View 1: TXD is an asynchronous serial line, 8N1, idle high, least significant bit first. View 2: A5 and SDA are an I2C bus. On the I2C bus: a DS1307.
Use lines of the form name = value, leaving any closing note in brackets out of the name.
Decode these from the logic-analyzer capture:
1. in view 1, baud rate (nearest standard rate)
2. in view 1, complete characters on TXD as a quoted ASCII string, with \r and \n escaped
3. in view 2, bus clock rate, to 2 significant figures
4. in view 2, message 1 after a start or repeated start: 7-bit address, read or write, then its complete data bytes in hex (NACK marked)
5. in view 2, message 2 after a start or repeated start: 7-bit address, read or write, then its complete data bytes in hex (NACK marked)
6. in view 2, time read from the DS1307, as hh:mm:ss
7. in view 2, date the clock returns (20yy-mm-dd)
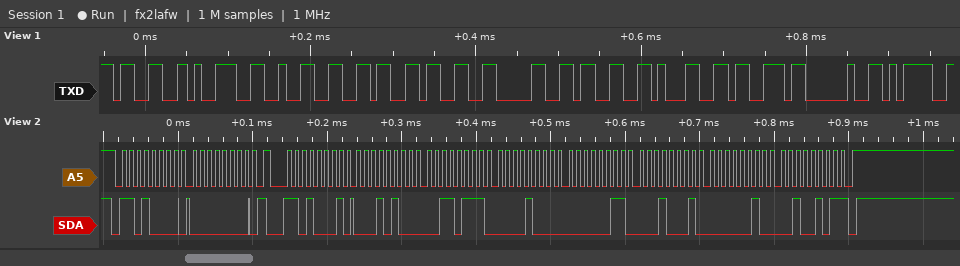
in view 1, baud rate = 115200 baud
in view 1, complete characters on TXD as a quoted ASCII string, with \r and \n escaped = "39263031s ="
in view 2, bus clock rate, to 2 significant figures = 100 kHz
in view 2, message 1 after a start or repeated start: 7-bit address, read or write, then its complete data bytes in hex = 0x68 write: 00
in view 2, message 2 after a start or repeated start: 7-bit address, read or write, then its complete data bytes in hex = 0x68 read: 14 37 08 03 11 02 25 NACK
in view 2, time read from the DS1307, as hh:mm:ss = 08:37:14
in view 2, date the clock returns = 2025-02-11
